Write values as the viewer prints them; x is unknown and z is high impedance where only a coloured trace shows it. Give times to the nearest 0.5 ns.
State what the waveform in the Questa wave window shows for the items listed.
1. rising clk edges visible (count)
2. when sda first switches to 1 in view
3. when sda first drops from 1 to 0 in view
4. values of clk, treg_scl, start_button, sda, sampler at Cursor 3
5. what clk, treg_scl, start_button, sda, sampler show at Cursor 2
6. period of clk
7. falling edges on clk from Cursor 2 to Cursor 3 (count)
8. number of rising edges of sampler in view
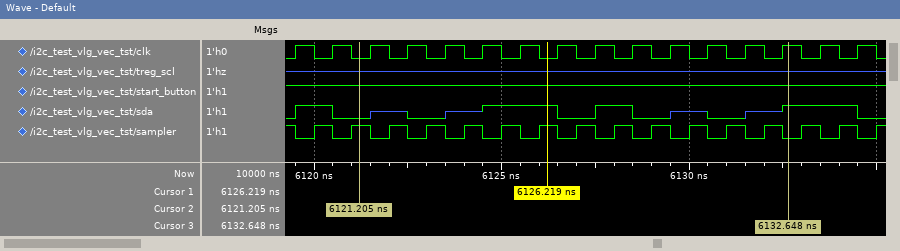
16
6119.5 ns
6120.5 ns
clk=1, treg_scl=z, start_button=1, sda=1, sampler=0
clk=0, treg_scl=z, start_button=1, sda=0, sampler=1
1 ns
11
16
